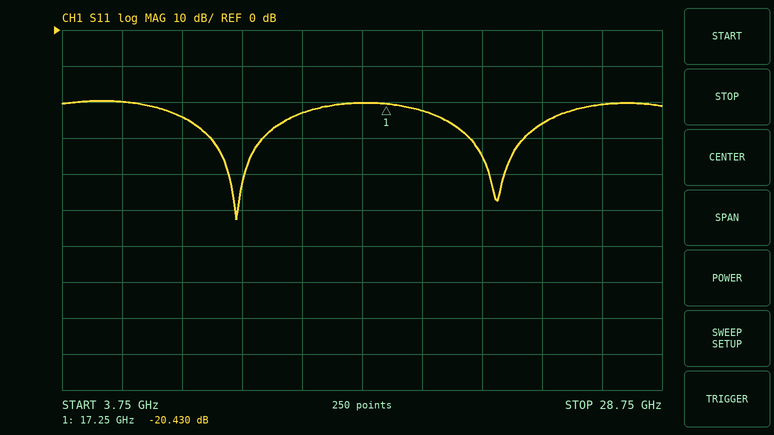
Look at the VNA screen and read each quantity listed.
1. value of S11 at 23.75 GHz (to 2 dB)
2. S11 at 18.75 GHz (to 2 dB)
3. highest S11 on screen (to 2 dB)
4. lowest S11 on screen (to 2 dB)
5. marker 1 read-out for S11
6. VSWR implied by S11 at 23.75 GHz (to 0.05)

-26 dB
-22 dB
-20 dB
-52 dB
-20.430 dB
1.10
